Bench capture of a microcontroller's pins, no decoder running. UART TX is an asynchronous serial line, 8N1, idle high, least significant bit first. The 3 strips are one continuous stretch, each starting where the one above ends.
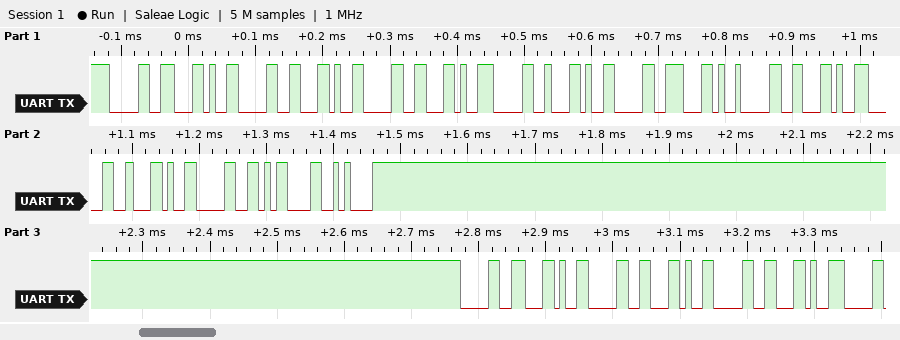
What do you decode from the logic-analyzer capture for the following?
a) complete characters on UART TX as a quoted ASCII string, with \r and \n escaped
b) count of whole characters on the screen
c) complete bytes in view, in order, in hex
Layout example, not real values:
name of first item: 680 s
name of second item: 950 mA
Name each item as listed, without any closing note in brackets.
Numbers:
complete characters on UART TX as a quoted ASCII string, with \r and \n escaped: "0,0,0,0,0,0,0,0\r\n0,0,0,"
count of whole characters on the screen: 23
complete bytes in view, in order, in hex: 30 2C 30 2C 30 2C 30 2C 30 2C 30 2C 30 2C 30 0D 0A 30 2C 30 2C 30 2C
